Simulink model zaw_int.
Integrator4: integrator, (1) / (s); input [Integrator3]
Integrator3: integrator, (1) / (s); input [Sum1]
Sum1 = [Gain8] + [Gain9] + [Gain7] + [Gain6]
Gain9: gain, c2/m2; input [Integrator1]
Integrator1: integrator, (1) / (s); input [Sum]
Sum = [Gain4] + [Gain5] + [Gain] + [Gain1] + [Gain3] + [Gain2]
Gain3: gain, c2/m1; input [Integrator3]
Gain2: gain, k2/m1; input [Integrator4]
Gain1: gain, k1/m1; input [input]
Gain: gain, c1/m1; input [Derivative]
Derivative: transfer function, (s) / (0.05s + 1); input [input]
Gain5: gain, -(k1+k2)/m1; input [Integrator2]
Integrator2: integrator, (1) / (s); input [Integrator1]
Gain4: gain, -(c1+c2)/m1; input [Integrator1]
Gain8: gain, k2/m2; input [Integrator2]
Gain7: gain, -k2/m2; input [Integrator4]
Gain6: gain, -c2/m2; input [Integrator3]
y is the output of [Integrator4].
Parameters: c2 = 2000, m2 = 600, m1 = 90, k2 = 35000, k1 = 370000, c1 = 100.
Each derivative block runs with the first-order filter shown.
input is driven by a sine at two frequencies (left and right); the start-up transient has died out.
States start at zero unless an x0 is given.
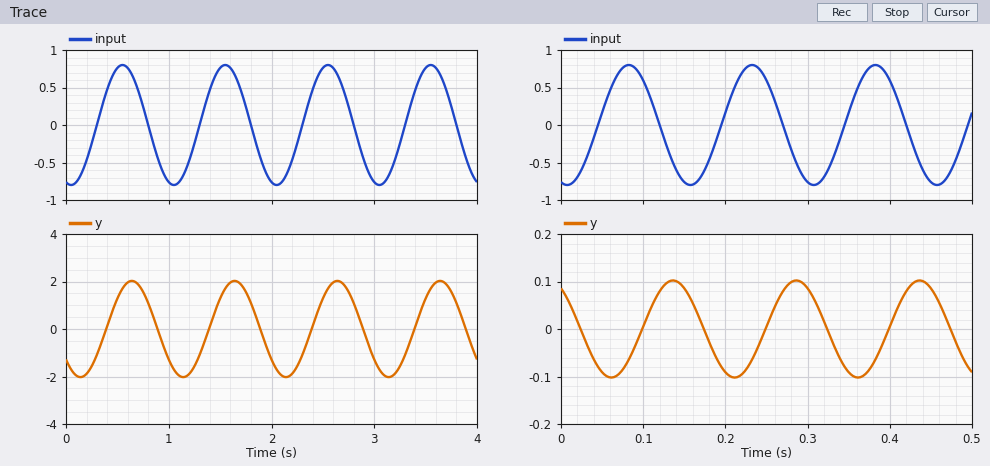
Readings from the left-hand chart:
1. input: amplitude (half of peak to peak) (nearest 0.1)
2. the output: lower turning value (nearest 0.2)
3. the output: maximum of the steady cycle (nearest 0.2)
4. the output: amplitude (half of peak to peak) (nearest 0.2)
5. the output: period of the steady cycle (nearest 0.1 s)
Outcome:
0.8
-2.0
2.0
2.0
1.0 s
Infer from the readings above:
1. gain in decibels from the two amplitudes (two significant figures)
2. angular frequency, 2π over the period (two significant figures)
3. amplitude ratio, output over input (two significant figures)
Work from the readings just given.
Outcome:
8.0 dB
6.3 rad/s
2.5
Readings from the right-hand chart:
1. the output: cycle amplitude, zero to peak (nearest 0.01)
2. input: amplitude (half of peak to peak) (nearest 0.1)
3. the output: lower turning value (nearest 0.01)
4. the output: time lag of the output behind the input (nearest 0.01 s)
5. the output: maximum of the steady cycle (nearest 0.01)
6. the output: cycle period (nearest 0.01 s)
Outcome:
0.10
0.8
-0.10
0.05 s
0.10
0.15 s
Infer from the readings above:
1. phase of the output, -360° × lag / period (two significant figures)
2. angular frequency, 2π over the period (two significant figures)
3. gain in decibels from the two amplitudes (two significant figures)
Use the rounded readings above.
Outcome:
-120°
42 rad/s
-18 dB
